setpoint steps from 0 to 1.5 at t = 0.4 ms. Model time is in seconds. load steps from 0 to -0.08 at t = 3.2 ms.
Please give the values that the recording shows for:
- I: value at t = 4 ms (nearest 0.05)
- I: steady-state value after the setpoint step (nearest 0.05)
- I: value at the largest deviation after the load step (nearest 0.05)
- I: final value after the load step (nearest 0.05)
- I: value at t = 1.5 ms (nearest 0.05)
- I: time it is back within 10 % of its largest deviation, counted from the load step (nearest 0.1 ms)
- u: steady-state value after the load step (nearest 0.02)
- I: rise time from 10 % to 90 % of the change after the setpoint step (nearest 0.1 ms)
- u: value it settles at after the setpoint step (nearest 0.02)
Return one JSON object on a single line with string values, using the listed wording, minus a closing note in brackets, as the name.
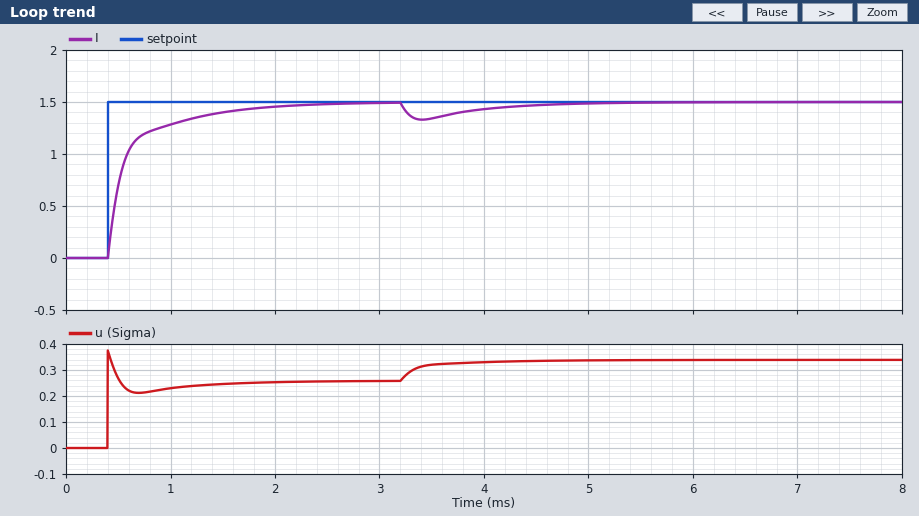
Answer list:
{"I: value at t = 4 ms": "1.45", "I: steady-state value after the setpoint step": "1.50", "I: value at the largest deviation after the load step": "1.35", "I: final value after the load step": "1.50", "I: value at t = 1.5 ms": "1.40", "I: time it is back within 10 % of its largest deviation, counted from the load step": "1.7 ms", "u: steady-state value after the load step": "0.34", "I: rise time from 10 % to 90 % of the change after the setpoint step": "0.8 ms", "u: value it settles at after the setpoint step": "0.26"}
